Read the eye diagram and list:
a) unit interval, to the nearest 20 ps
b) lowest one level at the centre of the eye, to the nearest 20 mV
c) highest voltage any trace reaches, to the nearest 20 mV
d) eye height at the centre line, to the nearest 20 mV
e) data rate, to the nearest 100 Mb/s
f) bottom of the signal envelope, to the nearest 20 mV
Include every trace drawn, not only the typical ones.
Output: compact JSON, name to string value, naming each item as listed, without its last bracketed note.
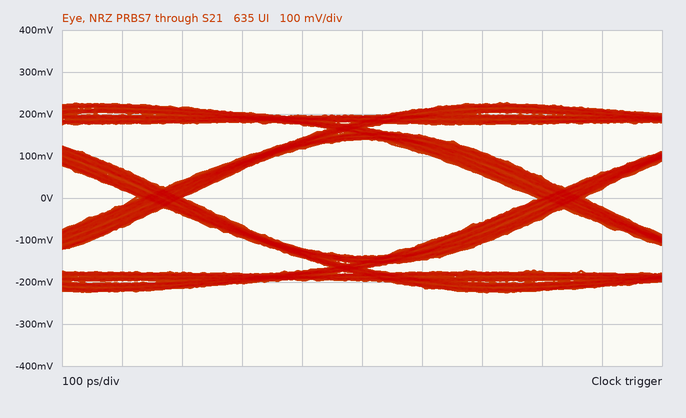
{"unit interval, to the nearest 20 ps": "660 ps", "lowest one level at the centre of the eye, to the nearest 20 mV": "140 mV", "highest voltage any trace reaches, to the nearest 20 mV": "220 mV", "eye height at the centre line, to the nearest 20 mV": "280 mV", "data rate, to the nearest 100 Mb/s": "1.5 Gb/s", "bottom of the signal envelope, to the nearest 20 mV": "-220 mV"}
